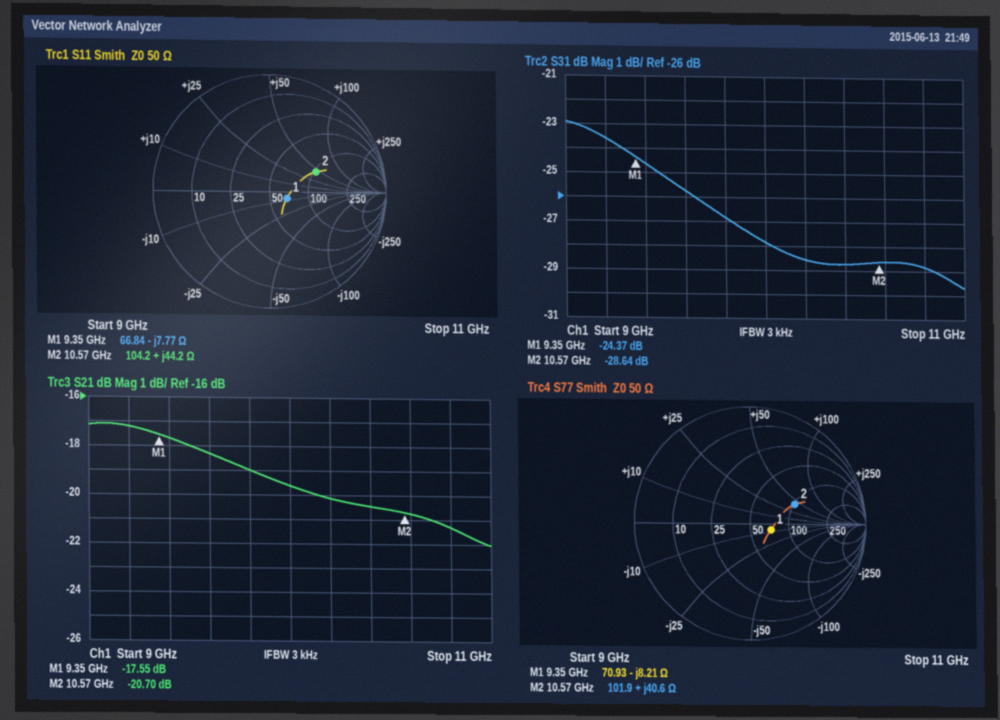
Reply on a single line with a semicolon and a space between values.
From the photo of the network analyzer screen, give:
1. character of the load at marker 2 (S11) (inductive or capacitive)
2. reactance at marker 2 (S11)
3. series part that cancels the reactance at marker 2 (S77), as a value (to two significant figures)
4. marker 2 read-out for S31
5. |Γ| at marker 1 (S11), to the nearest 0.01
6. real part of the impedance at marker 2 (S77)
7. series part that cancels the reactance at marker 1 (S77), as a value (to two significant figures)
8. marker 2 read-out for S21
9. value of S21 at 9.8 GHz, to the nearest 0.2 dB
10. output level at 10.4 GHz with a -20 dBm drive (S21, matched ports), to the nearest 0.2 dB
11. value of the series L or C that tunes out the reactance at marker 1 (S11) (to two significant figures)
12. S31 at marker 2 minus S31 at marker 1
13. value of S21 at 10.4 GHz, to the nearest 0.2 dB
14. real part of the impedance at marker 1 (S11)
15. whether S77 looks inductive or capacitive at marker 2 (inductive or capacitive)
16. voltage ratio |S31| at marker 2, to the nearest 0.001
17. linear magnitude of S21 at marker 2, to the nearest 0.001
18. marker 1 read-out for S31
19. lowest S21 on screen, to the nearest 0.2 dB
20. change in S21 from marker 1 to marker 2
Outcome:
inductive; +44.2 Ω; 370 fF; -28.64 dB; 0.16; 101.9 Ω; 140 pH; -20.70 dB; -19.0 dB; -40.4 dBm; 130 pH; -4.27 dB; -20.4 dB; 66.84 Ω; inductive; 0.037; 0.092; -24.37 dB; -22.0 dB; -3.15 dB
